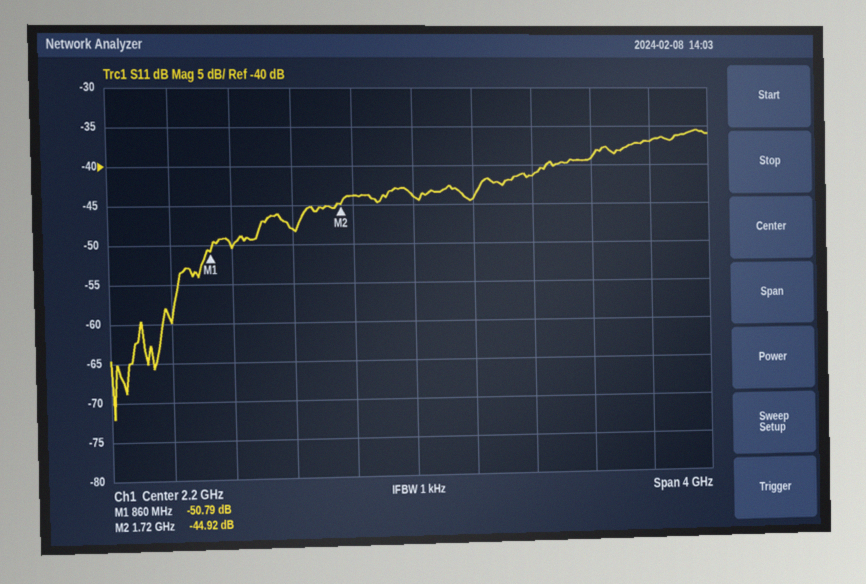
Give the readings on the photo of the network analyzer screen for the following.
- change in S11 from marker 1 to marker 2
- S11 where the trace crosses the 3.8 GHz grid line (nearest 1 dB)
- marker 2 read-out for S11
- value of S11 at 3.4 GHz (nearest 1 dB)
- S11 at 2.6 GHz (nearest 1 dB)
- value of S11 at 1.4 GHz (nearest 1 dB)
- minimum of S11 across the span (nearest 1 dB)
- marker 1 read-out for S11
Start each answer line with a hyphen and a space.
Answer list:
- 5.87 dB
- -37 dB
- -44.92 dB
- -39 dB
- -44 dB
- -48 dB
- -72 dB
- -50.79 dB
